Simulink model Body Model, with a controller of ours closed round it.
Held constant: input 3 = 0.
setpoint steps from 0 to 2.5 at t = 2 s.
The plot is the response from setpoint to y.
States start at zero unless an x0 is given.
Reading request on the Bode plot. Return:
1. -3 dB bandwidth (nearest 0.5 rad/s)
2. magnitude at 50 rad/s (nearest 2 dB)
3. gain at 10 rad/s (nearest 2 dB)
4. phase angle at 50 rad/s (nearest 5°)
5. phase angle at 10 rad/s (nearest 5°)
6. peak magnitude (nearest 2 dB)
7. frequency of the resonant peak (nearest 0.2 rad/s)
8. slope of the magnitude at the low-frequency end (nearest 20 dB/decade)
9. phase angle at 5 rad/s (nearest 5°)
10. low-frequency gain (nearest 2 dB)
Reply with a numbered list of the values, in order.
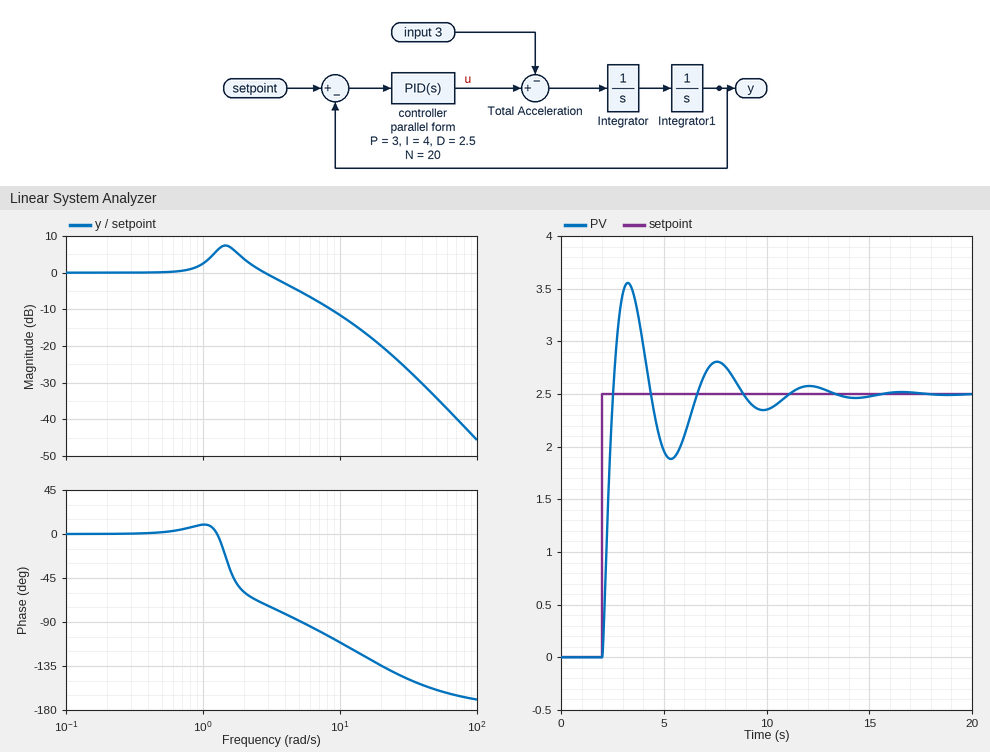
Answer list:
1. 4.0 rad/s
2. -34 dB
3. -12 dB
4. -160°
5. -110°
6. 8 dB
7. 1.4 rad/s
8. 0 dB/decade
9. -90°
10. 0 dB
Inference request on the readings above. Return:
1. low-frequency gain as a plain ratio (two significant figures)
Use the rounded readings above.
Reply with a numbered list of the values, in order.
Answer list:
1. 1.0
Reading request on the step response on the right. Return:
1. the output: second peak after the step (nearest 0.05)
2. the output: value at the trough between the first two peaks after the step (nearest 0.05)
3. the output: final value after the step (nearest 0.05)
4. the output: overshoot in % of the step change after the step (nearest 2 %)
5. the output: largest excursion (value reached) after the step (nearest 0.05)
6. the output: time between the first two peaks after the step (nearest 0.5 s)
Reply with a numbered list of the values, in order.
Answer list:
1. 2.80
2. 1.90
3. 2.50
4. 42 %
5. 3.55
6. 4.5 s
